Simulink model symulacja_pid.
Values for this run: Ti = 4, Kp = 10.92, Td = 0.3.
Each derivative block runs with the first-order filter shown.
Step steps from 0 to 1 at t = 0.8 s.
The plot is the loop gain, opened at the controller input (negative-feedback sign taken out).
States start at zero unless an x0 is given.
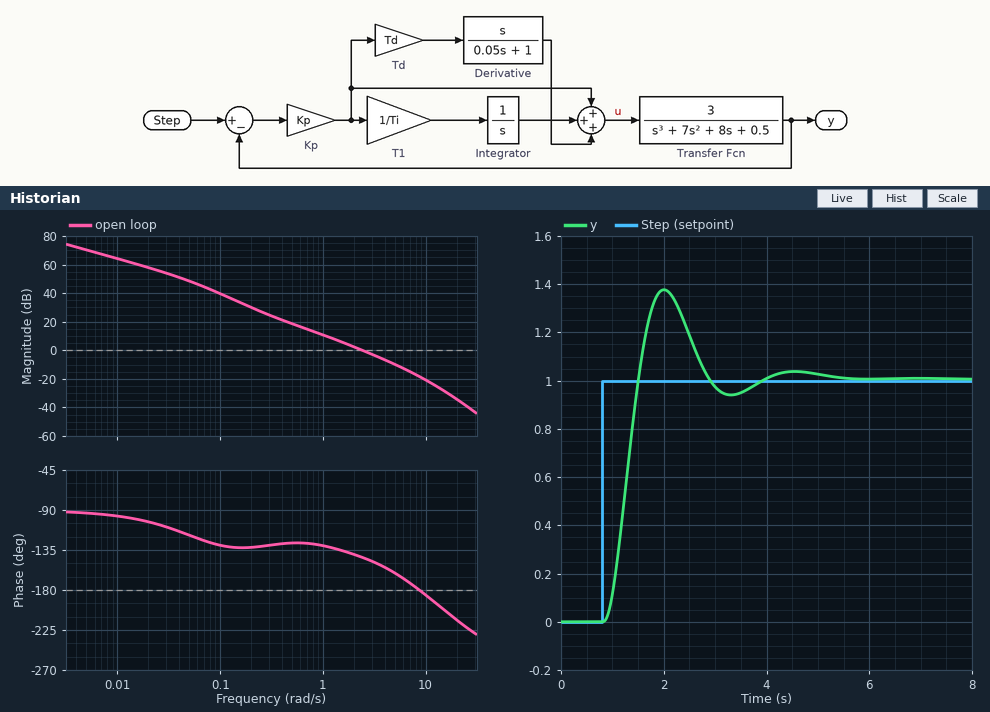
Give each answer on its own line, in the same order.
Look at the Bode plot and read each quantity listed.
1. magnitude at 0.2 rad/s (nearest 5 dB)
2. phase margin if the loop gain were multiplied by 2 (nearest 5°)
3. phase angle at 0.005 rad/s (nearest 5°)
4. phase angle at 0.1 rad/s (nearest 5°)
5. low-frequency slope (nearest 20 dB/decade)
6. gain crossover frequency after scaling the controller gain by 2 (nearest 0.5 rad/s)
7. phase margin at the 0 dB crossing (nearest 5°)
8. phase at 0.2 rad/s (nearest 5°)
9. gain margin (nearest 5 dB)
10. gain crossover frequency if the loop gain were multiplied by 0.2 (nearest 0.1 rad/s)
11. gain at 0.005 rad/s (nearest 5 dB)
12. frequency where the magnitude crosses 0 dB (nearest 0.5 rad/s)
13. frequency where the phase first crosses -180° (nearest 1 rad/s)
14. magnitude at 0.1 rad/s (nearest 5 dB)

30 dB
25°
-95°
-130°
-20 dB/decade
4.0 rad/s
35°
-130°
20 dB
0.8 rad/s
70 dB
2.5 rad/s
9 rad/s
40 dB
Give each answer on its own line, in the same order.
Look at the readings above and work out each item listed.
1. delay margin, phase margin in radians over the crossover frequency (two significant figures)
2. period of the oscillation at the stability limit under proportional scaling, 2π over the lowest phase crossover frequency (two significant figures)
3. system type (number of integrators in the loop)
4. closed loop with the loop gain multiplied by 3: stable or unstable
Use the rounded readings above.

0.24 s
0.70 s
1
stable
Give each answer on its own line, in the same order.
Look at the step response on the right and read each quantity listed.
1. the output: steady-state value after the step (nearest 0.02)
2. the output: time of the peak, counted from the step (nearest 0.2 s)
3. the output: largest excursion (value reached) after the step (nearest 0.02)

1.00
1.2 s
1.38
